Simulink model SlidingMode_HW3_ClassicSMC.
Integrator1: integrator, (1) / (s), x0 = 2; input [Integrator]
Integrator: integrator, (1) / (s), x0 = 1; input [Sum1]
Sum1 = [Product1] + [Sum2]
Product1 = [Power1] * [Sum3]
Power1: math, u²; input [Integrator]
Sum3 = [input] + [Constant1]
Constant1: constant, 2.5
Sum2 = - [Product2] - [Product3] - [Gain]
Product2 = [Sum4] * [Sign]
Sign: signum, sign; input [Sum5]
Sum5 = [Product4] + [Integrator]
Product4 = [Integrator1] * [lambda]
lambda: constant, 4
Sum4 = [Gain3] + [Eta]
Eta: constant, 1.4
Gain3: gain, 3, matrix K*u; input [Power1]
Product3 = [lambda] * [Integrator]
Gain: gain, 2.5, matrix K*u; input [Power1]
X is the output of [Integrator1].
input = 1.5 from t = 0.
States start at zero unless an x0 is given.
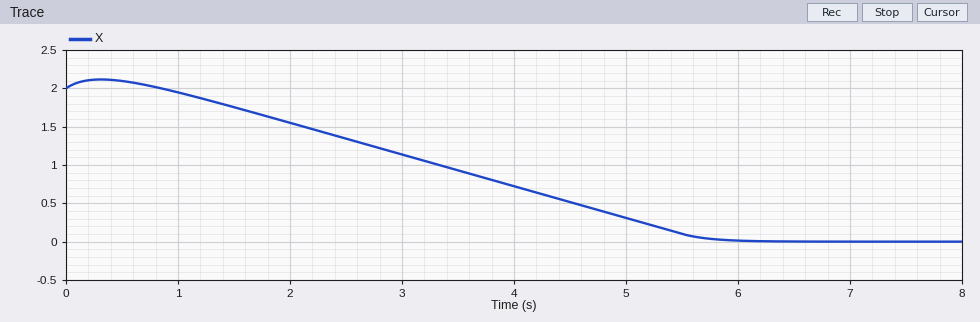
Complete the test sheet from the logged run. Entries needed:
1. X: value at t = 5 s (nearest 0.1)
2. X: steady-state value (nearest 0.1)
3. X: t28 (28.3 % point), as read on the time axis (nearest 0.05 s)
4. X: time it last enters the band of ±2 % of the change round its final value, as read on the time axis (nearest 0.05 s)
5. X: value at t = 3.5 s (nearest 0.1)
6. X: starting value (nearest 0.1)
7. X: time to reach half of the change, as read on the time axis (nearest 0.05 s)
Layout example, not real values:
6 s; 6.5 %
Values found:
0.3; 0.0; 2.30 s; 5.75 s; 0.9; 2.0; 3.35 s
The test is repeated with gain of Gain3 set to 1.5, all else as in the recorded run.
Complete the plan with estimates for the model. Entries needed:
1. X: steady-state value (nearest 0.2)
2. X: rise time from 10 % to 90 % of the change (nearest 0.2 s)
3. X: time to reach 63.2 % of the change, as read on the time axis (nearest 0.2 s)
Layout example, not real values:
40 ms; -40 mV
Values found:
0.0; 4.6 s; 4.6 s
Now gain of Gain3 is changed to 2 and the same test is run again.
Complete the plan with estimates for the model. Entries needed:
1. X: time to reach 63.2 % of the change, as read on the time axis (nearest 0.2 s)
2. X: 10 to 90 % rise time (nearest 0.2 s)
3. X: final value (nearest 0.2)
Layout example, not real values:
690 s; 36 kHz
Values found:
4.4 s; 4.4 s; 0.0
